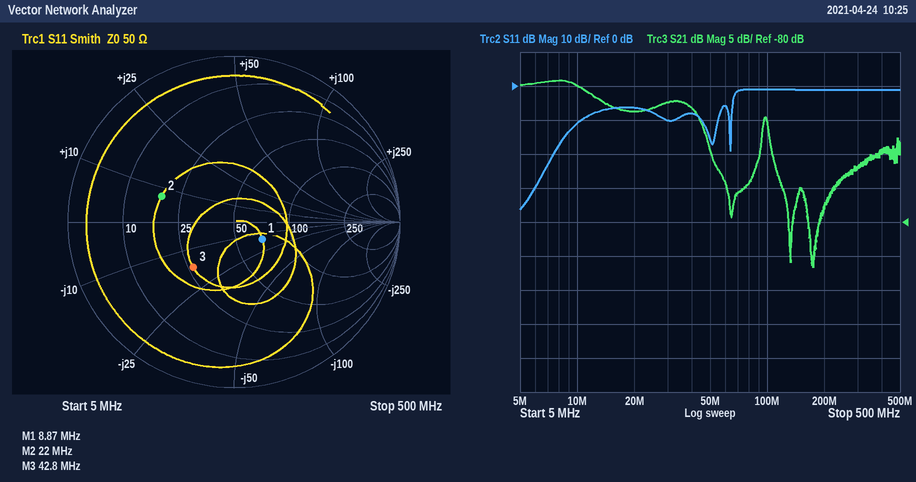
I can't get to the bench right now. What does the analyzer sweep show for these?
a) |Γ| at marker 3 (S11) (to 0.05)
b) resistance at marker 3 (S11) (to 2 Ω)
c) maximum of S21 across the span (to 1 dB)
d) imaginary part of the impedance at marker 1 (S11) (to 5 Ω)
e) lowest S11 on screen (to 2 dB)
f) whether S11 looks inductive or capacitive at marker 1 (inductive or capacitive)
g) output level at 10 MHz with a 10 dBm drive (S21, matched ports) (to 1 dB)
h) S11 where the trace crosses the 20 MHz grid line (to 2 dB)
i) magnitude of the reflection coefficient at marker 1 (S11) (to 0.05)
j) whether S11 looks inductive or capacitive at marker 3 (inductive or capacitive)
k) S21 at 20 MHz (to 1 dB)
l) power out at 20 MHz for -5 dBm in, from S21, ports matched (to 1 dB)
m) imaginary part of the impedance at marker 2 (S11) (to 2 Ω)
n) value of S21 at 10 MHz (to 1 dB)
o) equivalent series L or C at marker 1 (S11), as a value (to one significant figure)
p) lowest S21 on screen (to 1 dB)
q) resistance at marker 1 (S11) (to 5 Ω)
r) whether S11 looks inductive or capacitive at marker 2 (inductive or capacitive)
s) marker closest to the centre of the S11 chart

0.35
26 Ω
-59 dB
-15 Ω
-36 dB
capacitive
-50 dBm
-6 dB
0.20
capacitive
-64 dB
-69 dBm
+8 Ω
-60 dB
1 nF
-87 dB
70 Ω
inductive
marker 1
